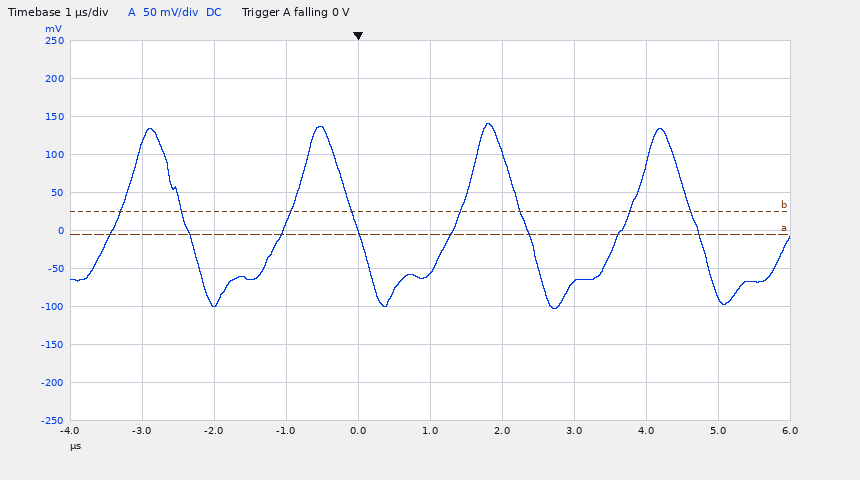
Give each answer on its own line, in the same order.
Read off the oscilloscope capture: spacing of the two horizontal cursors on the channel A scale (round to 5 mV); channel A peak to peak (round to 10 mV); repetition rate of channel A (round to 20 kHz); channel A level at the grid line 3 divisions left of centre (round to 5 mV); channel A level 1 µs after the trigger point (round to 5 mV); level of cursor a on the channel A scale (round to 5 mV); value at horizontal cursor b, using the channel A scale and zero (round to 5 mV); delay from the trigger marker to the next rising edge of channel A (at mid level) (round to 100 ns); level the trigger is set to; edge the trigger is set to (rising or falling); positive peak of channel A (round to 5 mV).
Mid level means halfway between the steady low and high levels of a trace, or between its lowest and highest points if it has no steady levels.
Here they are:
30 mV
240 mV
420 kHz
-100 mV
-55 mV
-5 mV
25 mV
1.4 µs
0 V
falling
140 mV
